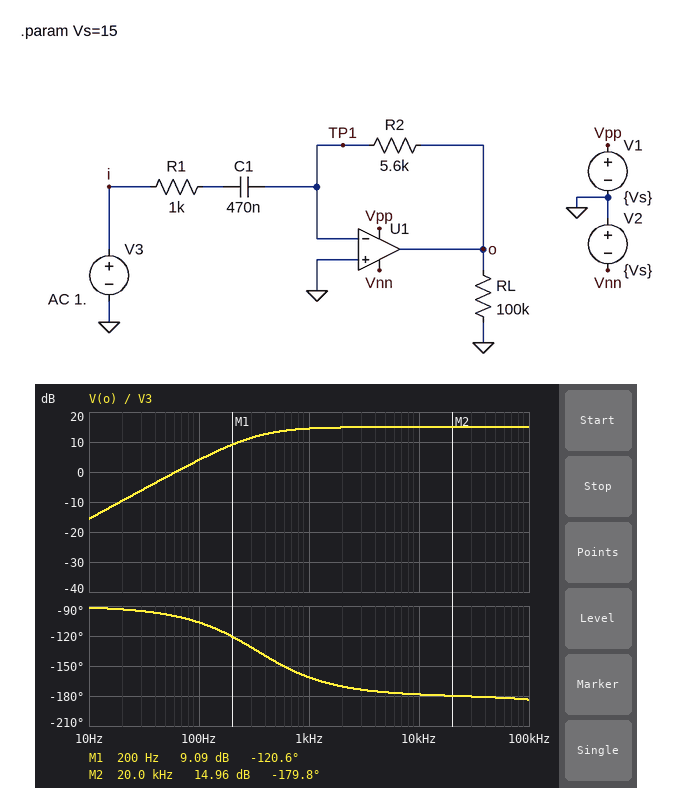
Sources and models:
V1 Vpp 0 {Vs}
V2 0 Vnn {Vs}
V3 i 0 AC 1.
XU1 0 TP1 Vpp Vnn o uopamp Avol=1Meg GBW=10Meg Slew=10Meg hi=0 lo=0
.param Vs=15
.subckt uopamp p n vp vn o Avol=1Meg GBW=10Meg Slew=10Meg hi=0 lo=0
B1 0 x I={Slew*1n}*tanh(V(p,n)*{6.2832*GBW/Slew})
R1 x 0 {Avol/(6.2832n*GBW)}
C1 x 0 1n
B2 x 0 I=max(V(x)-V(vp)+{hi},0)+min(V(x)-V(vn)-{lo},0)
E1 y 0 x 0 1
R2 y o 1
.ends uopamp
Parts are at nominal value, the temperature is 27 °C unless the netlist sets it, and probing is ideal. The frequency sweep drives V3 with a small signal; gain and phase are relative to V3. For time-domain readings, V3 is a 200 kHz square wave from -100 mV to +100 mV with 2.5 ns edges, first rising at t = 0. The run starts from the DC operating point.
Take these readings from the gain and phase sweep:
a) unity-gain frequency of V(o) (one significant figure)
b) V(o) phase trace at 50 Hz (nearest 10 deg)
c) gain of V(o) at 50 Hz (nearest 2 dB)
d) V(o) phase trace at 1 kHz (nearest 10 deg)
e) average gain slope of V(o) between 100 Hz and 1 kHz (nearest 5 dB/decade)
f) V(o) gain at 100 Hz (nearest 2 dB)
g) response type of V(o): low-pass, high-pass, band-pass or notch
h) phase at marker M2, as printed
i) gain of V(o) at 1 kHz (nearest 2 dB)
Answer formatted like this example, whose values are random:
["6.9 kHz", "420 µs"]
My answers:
["60 Hz", "-100 deg", "-2 dB", "-160 deg", "10 dB/decade", "4 dB", "high-pass", "-179.8 deg", "14 dB"]
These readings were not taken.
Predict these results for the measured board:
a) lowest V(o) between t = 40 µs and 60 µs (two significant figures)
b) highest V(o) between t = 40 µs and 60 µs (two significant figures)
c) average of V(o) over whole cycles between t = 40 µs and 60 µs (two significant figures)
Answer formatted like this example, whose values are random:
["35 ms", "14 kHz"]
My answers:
["-1.1 V", "67 mV", "-500 mV"]
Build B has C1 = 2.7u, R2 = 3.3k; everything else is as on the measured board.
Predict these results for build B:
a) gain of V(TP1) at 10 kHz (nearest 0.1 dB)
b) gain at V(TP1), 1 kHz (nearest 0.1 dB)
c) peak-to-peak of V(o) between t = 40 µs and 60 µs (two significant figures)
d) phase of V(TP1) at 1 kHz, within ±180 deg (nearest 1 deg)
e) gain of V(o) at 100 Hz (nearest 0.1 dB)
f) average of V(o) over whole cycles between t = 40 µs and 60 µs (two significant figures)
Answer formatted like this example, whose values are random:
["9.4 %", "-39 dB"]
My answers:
["-49.6 dB", "-69.6 dB", "660 mV", "93 deg", "9.1 dB", "-320 mV"]
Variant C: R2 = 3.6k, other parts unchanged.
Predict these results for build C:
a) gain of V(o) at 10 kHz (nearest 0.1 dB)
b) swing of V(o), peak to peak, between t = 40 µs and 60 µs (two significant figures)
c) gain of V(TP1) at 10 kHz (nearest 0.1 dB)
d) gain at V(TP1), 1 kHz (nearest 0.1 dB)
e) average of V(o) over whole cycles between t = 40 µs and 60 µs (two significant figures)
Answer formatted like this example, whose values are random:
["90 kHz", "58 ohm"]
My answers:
["11.1 dB", "730 mV", "-48.9 dB", "-69.3 dB", "-320 mV"]
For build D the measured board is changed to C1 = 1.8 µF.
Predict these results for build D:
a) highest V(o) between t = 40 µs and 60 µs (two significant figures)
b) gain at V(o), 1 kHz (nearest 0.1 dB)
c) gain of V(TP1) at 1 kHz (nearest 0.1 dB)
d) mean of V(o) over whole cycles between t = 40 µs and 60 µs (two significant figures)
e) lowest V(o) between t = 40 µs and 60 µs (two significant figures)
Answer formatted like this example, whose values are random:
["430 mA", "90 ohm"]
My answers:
["18 mV", "14.9 dB", "-65.1 dB", "-540 mV", "-1.1 V"]
